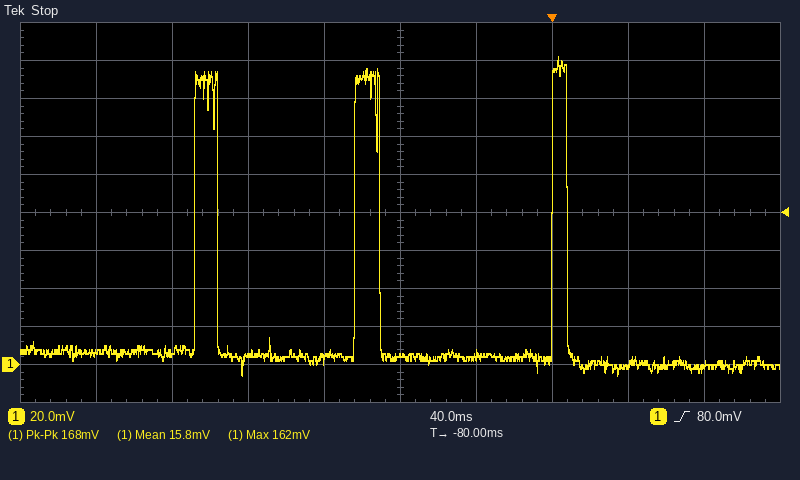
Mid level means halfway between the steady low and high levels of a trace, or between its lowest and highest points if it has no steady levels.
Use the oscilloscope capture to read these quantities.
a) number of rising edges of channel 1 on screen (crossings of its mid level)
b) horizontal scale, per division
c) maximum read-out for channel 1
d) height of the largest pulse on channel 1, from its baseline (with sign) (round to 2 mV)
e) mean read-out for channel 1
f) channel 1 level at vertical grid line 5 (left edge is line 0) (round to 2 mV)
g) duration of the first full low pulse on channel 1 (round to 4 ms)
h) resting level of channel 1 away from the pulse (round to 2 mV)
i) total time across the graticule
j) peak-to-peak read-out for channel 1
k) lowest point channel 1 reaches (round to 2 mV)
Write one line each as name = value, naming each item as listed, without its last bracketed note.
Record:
number of rising edges of channel 1 on screen = 3
horizontal scale, per division = 40 ms
maximum read-out for channel 1 = 162 mV
height of the largest pulse on channel 1, from its baseline (with sign) = +158 mV
mean read-out for channel 1 = 15.8 mV
channel 1 level at vertical grid line 5 (left edge is line 0) = 4 mV
duration of the first full low pulse on channel 1 = 72 ms
resting level of channel 1 away from the pulse = 4 mV
total time across the graticule = 400 ms
peak-to-peak read-out for channel 1 = 168 mV
lowest point channel 1 reaches = -6 mV
